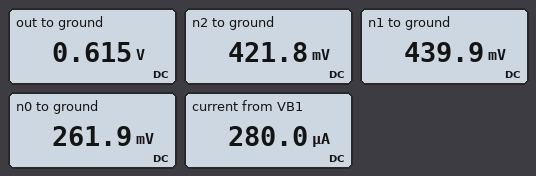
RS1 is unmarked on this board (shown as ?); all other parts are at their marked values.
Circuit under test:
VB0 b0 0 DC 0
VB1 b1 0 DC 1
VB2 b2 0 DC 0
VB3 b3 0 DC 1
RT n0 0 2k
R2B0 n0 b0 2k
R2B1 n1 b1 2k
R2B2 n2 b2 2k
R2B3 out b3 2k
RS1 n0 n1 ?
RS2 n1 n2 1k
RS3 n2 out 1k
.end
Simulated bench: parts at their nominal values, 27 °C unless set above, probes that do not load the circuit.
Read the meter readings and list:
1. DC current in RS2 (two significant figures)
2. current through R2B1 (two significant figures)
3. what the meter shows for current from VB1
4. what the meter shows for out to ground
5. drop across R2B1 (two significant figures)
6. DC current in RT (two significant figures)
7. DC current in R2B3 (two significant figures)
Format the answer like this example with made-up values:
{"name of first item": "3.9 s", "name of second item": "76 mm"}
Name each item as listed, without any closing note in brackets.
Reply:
{"DC current in RS2": "18 µA", "current through R2B1": "280 µA", "what the meter shows for current from VB1": "280.0 µA", "what the meter shows for out to ground": "0.615 V", "drop across R2B1": "560 mV", "DC current in RT": "130 µA", "DC current in R2B3": "190 µA"}
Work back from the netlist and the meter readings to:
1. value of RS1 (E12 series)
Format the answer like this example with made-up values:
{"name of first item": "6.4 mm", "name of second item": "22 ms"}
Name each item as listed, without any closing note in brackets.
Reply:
{"value of RS1": "680 Ω"}
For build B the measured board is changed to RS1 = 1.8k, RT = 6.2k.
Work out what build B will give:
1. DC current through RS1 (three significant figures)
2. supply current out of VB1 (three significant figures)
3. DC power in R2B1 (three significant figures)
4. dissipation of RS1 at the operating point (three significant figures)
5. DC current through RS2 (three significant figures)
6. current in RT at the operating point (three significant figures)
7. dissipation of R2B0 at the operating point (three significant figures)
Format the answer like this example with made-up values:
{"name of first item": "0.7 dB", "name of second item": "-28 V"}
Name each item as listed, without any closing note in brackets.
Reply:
{"DC current through RS1": "164 µA", "supply current out of VB1": "229 µA", "DC power in R2B1": "105 µW", "dissipation of RS1 at the operating point": "48.3 µW", "DC current through RS2": "64.8 µA", "current in RT at the operating point": "40.0 µA", "dissipation of R2B0 at the operating point": "30.7 µW"}
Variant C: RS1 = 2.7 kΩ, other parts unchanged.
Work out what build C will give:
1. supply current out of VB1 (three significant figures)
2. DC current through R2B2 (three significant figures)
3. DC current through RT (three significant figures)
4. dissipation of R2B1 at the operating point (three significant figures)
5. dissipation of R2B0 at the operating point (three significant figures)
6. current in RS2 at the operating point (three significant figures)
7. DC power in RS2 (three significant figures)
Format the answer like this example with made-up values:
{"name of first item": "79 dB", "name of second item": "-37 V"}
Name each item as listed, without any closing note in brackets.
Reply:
{"supply current out of VB1": "222 µA", "DC current through R2B2": "243 µA", "DC current through RT": "75.2 µA", "dissipation of R2B1 at the operating point": "98.3 µW", "dissipation of R2B0 at the operating point": "11.3 µW", "current in RS2 at the operating point": "71.2 µA", "DC power in RS2": "5.07 µW"}
